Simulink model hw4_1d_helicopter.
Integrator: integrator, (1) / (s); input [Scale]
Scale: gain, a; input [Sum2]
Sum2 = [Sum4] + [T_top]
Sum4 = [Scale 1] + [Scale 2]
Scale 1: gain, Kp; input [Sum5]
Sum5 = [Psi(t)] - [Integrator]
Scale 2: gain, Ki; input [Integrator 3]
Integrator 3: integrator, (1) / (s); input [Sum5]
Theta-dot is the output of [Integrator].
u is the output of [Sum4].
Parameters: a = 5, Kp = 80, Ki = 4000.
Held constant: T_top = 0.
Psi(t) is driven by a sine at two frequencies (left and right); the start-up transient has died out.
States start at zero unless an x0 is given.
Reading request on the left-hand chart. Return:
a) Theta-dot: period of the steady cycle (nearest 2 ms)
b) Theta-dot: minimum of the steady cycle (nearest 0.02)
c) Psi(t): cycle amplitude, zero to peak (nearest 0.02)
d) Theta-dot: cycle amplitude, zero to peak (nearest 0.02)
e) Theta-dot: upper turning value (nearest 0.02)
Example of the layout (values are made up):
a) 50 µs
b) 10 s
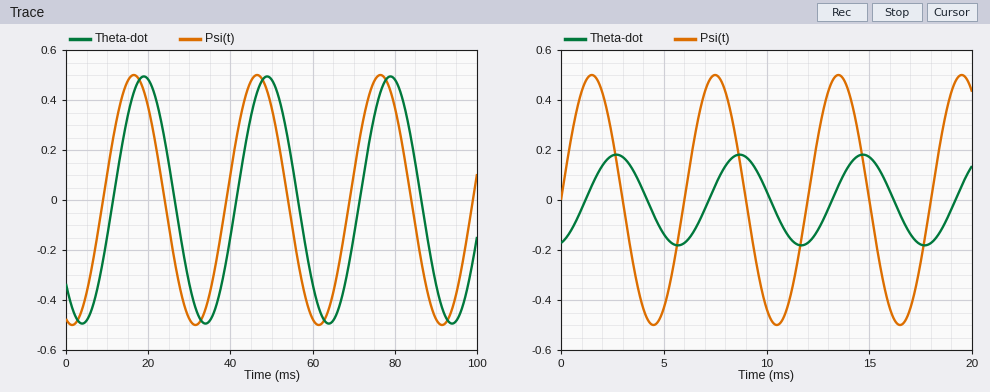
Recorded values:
a) 30 ms
b) -0.50
c) 0.50
d) 0.50
e) 0.50
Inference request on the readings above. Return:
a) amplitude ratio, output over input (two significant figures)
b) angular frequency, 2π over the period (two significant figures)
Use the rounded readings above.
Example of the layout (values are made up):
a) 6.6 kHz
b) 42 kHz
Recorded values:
a) 1.0
b) 0.21 rad/ms
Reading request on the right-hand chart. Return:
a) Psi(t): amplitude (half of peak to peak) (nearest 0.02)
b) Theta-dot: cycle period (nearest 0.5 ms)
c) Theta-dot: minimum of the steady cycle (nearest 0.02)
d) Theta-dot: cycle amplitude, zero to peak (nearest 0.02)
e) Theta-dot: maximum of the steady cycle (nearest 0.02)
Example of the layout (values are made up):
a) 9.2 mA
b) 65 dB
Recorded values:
a) 0.50
b) 6.0 ms
c) -0.18
d) 0.18
e) 0.18
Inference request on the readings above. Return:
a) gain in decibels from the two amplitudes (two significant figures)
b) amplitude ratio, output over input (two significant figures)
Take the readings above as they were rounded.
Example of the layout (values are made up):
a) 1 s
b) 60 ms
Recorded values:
a) -8.9 dB
b) 0.36
